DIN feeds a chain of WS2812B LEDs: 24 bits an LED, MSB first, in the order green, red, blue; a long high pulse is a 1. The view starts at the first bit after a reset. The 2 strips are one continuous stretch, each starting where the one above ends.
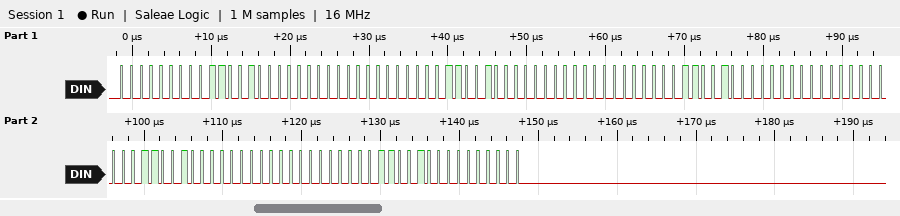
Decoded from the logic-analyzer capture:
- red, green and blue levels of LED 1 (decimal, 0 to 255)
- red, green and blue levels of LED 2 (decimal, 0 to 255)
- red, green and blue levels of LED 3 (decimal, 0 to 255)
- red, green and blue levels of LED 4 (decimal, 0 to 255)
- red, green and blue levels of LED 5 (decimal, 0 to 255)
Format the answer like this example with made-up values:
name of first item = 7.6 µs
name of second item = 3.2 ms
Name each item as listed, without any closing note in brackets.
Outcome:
red, green and blue levels of LED 1 = 100, 0, 0
red, green and blue levels of LED 2 = 100, 0, 0
red, green and blue levels of LED 3 = 100, 0, 0
red, green and blue levels of LED 4 = 100, 0, 0
red, green and blue levels of LED 5 = 100, 0, 0
